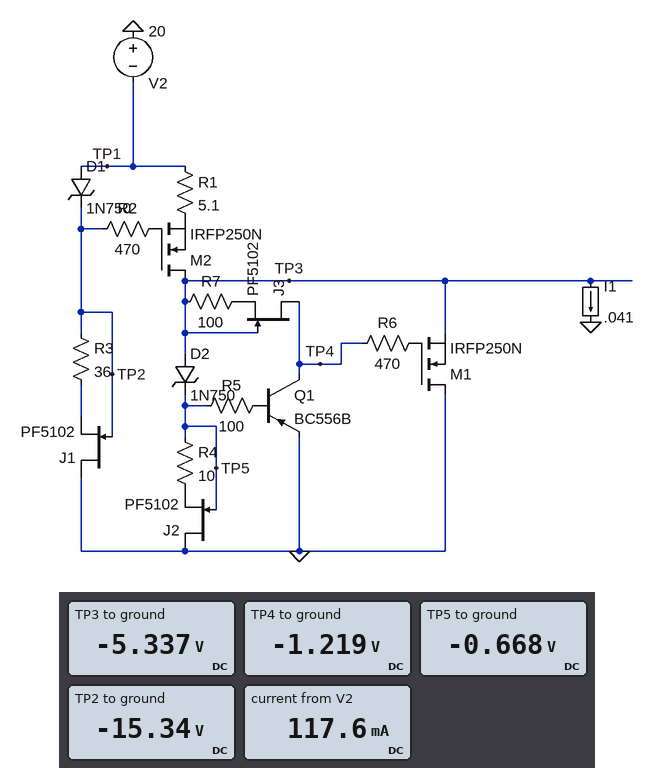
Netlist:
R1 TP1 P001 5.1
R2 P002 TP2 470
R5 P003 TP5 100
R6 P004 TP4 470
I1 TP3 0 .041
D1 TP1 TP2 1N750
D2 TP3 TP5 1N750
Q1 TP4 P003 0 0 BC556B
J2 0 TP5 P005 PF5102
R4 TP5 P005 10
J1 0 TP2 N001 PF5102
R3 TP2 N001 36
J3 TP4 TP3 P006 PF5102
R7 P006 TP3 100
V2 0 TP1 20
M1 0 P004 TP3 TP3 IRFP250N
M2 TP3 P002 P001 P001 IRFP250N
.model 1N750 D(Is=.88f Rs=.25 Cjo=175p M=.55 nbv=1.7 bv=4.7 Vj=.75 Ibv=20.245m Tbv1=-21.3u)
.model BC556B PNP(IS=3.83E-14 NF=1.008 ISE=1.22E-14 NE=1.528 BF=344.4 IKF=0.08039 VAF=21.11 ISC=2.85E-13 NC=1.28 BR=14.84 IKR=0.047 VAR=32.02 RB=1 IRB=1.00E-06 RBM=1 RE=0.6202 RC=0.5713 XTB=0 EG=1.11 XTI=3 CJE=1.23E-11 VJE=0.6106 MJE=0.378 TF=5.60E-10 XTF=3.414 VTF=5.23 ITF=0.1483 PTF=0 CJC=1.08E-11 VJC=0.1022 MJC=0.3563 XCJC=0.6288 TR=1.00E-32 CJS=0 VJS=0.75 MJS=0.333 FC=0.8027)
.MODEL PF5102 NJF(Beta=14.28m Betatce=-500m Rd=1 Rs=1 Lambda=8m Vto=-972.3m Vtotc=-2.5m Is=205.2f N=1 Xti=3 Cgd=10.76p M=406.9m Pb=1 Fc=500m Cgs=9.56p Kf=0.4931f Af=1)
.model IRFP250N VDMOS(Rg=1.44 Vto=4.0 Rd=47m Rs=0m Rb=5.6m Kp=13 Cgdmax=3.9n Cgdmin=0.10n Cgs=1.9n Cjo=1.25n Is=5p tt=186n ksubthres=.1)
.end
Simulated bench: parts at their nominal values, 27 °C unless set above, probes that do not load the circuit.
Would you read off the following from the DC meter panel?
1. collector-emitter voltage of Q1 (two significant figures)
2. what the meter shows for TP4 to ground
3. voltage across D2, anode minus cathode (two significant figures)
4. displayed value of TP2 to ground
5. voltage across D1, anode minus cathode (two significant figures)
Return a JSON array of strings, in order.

["-1.2 V", "-1.219 V", "-4.7 V", "-15.34 V", "-4.7 V"]
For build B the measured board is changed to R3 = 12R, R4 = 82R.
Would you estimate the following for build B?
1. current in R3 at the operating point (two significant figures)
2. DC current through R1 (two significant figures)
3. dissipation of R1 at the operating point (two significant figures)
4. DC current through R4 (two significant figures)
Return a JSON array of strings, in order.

["11 mA", "110 mA", "65 mW", "4.2 mA"]
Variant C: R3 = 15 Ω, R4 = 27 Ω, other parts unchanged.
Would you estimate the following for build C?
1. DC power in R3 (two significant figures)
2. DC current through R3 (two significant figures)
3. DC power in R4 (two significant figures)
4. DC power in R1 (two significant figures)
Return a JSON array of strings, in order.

["1.6 mW", "10 mA", "1.4 mW", "64 mW"]
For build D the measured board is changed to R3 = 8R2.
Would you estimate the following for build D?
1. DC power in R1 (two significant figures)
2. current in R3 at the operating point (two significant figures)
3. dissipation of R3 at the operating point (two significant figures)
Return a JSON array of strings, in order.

["66 mW", "12 mA", "1.2 mW"]
